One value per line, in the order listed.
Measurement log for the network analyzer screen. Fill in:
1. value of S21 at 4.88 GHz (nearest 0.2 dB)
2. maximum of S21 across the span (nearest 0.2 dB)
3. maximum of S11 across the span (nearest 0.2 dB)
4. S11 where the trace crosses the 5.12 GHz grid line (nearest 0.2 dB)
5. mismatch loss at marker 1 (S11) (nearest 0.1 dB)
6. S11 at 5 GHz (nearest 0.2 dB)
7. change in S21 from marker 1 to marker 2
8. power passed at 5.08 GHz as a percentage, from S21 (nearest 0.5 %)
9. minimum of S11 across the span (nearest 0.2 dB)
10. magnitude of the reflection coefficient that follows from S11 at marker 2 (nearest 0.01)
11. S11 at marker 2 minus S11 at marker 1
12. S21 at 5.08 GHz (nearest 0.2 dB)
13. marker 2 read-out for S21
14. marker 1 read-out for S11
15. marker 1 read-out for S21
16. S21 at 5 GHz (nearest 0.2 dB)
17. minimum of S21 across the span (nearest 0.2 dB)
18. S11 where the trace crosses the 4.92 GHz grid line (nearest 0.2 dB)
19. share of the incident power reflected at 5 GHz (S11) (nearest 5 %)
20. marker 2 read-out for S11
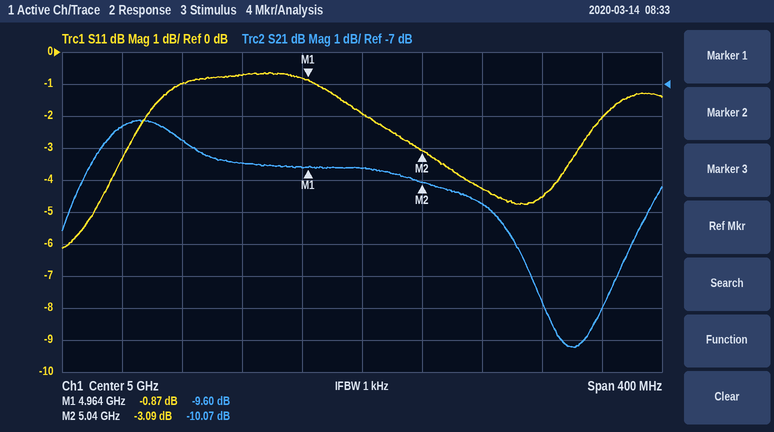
-8.8 dB
-8.2 dB
-0.6 dB
-4.6 dB
7.4 dB
-2.0 dB
-0.47 dB
8.5 %
-6.2 dB
0.70
-2.22 dB
-10.8 dB
-10.07 dB
-0.87 dB
-9.60 dB
-9.6 dB
-15.2 dB
-0.8 dB
65 %
-3.09 dB
